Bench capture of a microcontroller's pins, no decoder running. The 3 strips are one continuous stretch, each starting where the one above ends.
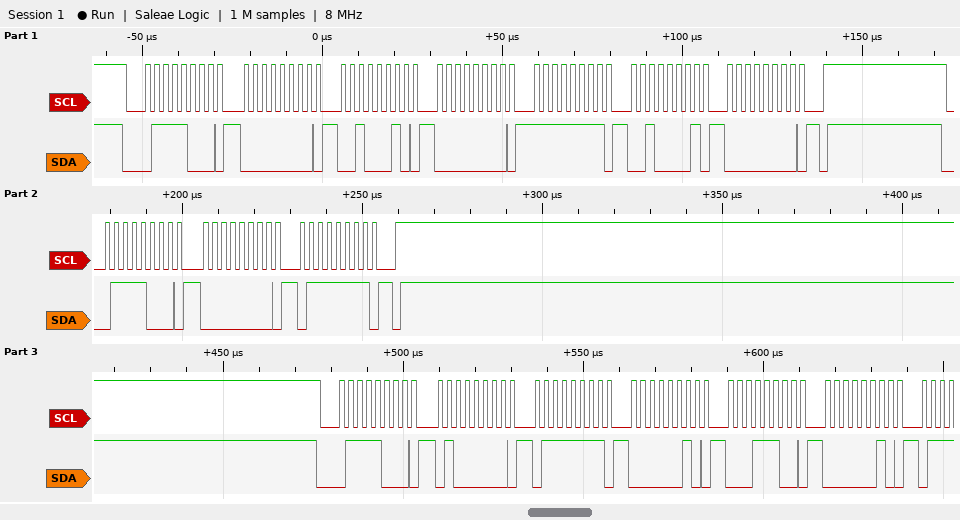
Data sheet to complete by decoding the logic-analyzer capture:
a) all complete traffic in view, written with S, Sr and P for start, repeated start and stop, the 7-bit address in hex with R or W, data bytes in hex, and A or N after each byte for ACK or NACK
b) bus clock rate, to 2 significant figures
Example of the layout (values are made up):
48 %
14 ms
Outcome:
S 3CW A 00 A 22 A 00 A FF A 21 A 00 A P S 3CW A 00 A 7F A P S 3CW A 40 A 7F A 02 A 1C A 02 A
400 kHz
